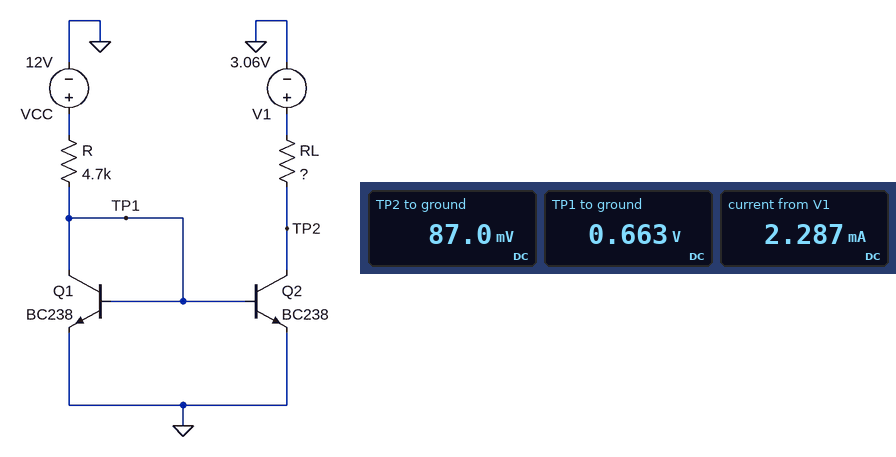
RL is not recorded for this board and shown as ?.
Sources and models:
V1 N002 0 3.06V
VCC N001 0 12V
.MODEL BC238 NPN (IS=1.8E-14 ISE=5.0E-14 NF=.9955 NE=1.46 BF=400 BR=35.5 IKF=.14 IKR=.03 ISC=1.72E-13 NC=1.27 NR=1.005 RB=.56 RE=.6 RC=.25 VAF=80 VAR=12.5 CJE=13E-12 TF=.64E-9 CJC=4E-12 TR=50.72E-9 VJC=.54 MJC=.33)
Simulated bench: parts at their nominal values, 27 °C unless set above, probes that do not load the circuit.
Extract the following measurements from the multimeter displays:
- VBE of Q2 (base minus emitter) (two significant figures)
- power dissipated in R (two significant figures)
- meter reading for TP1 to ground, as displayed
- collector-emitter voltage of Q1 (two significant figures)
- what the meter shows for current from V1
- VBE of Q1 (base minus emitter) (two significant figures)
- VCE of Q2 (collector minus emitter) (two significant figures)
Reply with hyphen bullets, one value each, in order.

- 660 mV
- 27 mW
- 0.663 V
- 660 mV
- 2.287 mA
- 660 mV
- 87 mV
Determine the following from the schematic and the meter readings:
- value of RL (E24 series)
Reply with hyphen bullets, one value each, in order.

- 1.3 kΩ
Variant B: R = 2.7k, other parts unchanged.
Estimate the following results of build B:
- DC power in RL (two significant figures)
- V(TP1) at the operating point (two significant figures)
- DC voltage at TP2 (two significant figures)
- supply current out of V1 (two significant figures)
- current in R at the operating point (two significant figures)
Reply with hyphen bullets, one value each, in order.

- 7.1 mW
- 680 mV
- 21 mV
- 2.3 mA
- 4.2 mA
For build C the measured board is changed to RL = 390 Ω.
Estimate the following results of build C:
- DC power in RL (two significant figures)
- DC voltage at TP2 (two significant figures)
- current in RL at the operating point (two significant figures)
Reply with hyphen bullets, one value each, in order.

- 2.3 mW
- 2.1 V
- 2.4 mA
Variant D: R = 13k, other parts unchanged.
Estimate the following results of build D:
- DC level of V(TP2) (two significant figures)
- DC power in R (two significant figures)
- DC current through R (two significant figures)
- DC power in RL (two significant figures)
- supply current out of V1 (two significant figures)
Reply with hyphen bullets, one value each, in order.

- 1.9 V
- 9.9 mW
- 870 µA
- 1.0 mW
- 880 µA
